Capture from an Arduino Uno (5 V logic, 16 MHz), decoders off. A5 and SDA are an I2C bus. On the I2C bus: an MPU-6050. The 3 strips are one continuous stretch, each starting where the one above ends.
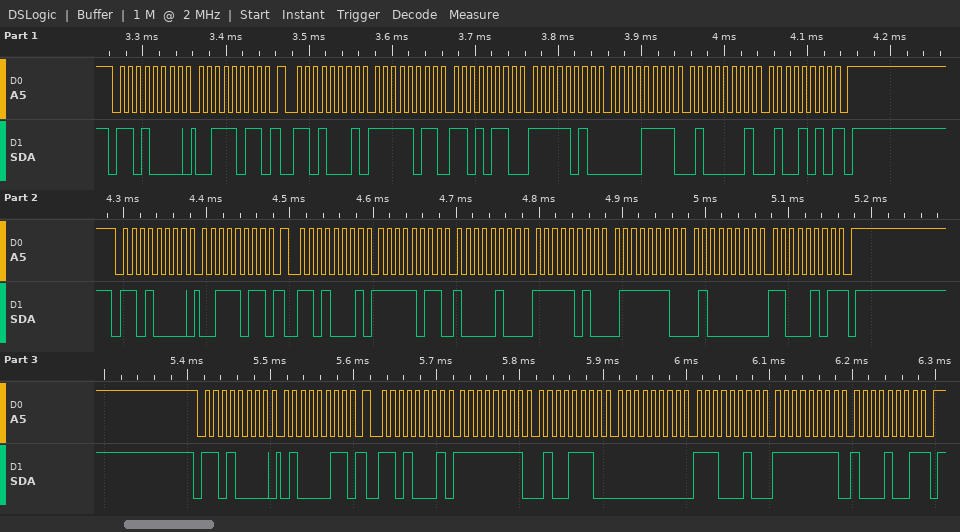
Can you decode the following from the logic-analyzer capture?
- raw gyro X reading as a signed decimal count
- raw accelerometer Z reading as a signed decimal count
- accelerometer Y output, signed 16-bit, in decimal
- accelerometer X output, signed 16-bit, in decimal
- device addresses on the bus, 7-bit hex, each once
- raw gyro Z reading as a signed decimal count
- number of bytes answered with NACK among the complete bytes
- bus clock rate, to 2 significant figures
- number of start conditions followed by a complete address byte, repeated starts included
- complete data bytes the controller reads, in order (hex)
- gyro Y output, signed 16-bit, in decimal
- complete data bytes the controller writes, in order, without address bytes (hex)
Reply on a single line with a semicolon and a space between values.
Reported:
-178; 16714; -1521; -1066; 0x68; -119; 3; 100 kHz; 6; FB D6 FA 0F 41 4A FB 84 FA 7E 40 C5 FF 4E 00 E2 FF 89; 226; 3B 3B 43
